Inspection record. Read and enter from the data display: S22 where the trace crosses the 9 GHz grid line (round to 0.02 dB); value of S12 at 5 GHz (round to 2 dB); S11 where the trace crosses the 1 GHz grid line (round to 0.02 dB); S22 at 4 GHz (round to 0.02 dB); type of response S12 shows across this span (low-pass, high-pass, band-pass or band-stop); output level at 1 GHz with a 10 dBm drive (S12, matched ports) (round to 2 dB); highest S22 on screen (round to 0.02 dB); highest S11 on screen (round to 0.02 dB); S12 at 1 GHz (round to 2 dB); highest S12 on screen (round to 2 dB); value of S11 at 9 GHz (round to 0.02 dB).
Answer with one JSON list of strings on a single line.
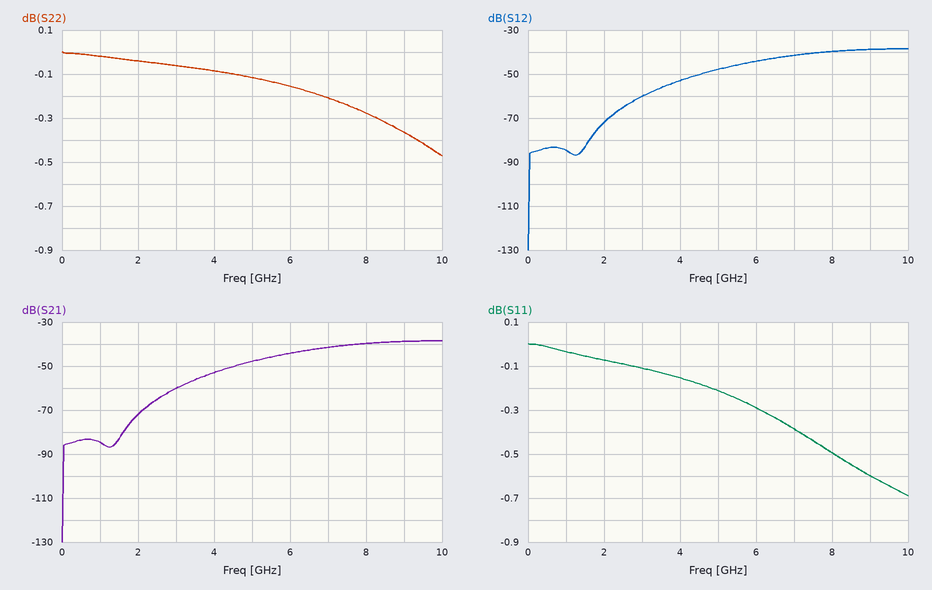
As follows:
["-0.36 dB", "-48 dB", "-0.04 dB", "-0.08 dB", "high-pass", "-74 dBm", "0.00 dB", "0.00 dB", "-84 dB", "-38 dB", "-0.60 dB"]
